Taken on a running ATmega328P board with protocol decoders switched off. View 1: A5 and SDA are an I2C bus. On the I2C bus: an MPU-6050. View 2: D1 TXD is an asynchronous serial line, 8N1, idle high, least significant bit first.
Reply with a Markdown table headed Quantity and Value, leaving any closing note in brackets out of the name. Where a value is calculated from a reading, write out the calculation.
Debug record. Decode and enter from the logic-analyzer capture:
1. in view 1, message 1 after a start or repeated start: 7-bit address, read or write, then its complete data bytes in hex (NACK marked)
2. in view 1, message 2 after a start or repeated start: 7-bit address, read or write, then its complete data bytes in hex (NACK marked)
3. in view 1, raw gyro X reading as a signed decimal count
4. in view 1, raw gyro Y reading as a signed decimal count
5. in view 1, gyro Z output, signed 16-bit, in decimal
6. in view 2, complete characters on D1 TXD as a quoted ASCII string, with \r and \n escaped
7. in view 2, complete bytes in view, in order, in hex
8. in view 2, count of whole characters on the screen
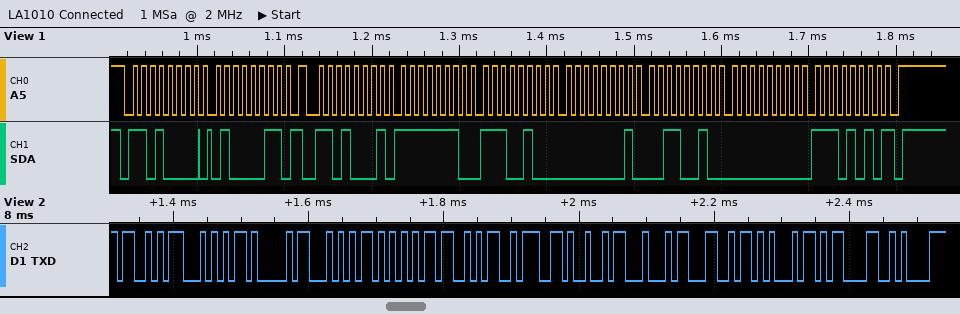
| Quantity | Value |
|---|---|
| in view 1, message 1 after a start or repeated start: 7-bit address, read or write, then its complete data bytes in hex | 0x68 write: 43 |
| in view 1, message 2 after a start or repeated start: 7-bit address, read or write, then its complete data bytes in hex | 0x68 read: FE E4 01 32 00 EA NACK |
| in view 1, raw gyro X reading as a signed decimal count | 0xFEE4 = -284 |
| in view 1, raw gyro Y reading as a signed decimal count | 0x0132 = 306 |
| in view 1, gyro Z output, signed 16-bit, in decimal | 0x00EA = 234 |
| in view 2, complete characters on D1 TXD as a quoted ASCII string, with \r and \n escaped | "STATUS:IDLE\r\n" |
| in view 2, complete bytes in view, in order, in hex | 53 54 41 54 55 53 3A 49 44 4C 45 0D 0A |
| in view 2, count of whole characters on the screen | 13 |
